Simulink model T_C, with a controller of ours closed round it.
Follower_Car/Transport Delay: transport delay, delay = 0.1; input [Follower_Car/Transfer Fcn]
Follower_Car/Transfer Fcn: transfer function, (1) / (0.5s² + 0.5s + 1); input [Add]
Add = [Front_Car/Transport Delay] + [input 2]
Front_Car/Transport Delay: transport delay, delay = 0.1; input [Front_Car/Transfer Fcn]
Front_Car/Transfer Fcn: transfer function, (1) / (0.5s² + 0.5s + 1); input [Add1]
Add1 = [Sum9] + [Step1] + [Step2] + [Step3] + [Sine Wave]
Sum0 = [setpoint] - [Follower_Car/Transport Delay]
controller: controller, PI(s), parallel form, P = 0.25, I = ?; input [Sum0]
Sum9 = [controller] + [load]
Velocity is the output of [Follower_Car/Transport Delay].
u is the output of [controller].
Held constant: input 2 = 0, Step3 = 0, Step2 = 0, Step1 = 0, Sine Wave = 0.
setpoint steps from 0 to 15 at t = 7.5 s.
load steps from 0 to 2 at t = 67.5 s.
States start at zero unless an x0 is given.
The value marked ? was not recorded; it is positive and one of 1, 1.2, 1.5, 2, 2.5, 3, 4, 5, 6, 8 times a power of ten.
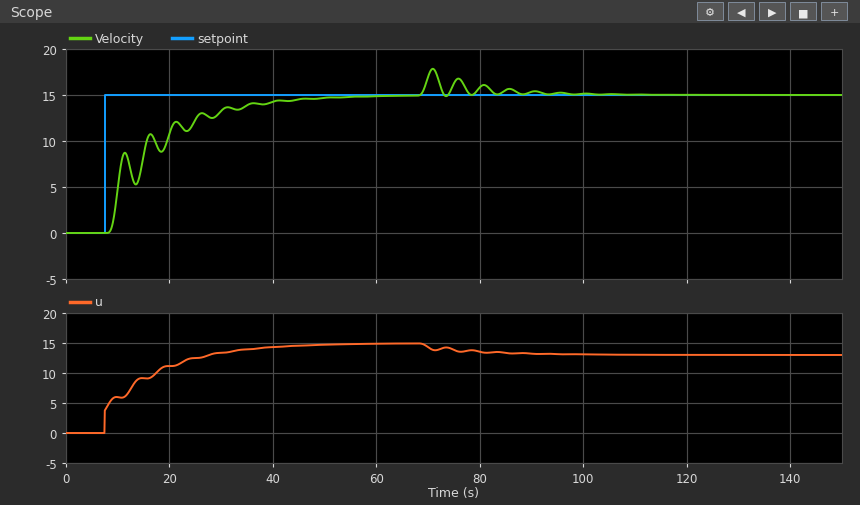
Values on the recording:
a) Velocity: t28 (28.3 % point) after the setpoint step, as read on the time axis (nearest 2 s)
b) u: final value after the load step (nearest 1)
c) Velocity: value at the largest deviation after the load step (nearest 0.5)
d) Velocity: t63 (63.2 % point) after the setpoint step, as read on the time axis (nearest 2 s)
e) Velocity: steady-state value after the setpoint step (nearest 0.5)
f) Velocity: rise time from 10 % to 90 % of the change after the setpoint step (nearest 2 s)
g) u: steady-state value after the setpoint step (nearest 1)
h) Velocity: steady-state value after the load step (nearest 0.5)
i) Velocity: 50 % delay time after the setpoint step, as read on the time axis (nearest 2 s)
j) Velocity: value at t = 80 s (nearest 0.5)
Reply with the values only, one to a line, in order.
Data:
10 s
13
18.0
16 s
15.0
22 s
15
15.0
10 s
16.0
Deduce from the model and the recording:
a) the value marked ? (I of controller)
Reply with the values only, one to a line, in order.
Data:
0.1
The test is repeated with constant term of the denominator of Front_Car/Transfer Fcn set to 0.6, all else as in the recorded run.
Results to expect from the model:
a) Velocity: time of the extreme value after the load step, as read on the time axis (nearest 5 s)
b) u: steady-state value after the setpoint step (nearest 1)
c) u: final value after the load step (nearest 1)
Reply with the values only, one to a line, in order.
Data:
70 s
9
7
